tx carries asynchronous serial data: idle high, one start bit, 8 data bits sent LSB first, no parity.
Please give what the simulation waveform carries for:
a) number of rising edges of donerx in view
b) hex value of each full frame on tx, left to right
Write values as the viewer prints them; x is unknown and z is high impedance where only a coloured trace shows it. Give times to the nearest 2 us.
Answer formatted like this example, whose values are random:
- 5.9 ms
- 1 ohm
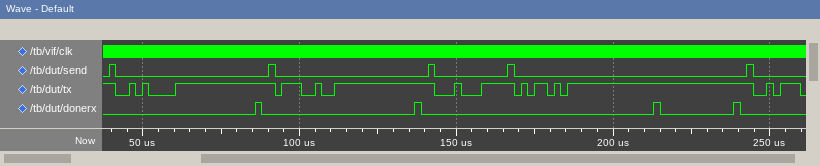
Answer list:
- 4
- 0A, 27, C4, AD
